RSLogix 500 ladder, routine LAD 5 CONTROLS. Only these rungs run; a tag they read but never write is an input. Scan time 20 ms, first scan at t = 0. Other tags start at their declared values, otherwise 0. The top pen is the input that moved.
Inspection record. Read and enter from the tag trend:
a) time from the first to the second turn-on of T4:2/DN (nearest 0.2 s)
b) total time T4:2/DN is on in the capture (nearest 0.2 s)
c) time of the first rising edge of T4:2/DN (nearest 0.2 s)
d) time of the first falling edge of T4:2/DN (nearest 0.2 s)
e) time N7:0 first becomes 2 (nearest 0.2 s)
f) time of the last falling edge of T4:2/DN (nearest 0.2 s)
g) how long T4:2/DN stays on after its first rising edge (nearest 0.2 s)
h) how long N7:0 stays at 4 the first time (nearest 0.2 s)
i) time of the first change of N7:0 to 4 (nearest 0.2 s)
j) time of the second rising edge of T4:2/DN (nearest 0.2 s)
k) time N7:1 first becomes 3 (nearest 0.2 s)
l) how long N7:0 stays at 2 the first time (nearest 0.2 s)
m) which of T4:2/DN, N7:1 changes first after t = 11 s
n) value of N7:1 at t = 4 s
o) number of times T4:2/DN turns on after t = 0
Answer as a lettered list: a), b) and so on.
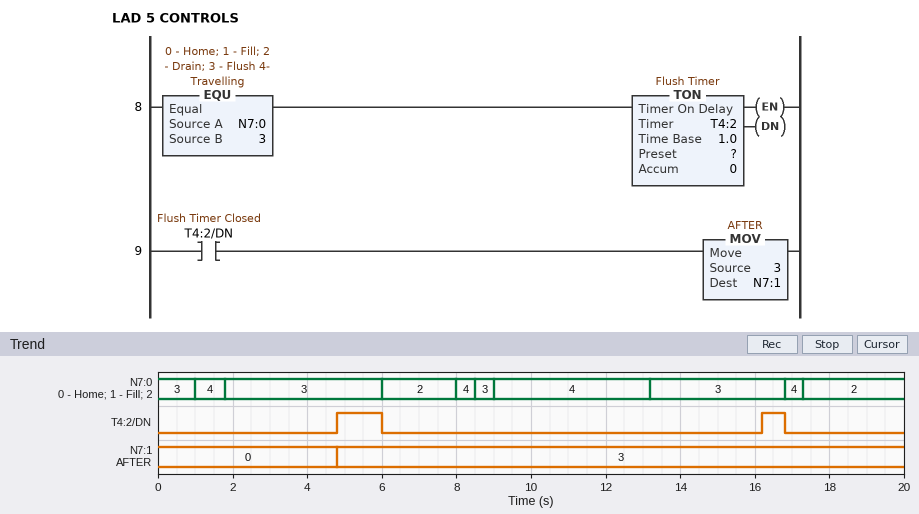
a) 11.4 s
b) 1.8 s
c) 4.8 s
d) 6.0 s
e) 6.0 s
f) 16.8 s
g) 1.2 s
h) 0.8 s
i) 1.0 s
j) 16.2 s
k) 4.8 s
l) 2.0 s
m) T4:2/DN
n) 0
o) 2
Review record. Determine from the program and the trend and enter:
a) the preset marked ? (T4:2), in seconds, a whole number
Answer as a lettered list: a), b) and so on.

a) 3 s
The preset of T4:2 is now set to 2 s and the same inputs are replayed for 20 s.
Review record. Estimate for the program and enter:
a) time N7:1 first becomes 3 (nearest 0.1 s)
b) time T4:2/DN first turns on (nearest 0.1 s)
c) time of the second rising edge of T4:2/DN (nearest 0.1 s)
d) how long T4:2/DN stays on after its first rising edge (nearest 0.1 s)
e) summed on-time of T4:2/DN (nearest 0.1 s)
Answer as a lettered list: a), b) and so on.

a) 3.8 s
b) 3.8 s
c) 15.2 s
d) 2.2 s
e) 3.8 s
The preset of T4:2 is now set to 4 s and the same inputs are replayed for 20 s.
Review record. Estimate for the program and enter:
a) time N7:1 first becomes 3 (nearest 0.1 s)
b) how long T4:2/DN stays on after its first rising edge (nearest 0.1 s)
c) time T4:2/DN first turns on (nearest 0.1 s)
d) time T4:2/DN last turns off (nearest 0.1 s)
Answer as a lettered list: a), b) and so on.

a) 5.8 s
b) 0.2 s
c) 5.8 s
d) 6.0 s
